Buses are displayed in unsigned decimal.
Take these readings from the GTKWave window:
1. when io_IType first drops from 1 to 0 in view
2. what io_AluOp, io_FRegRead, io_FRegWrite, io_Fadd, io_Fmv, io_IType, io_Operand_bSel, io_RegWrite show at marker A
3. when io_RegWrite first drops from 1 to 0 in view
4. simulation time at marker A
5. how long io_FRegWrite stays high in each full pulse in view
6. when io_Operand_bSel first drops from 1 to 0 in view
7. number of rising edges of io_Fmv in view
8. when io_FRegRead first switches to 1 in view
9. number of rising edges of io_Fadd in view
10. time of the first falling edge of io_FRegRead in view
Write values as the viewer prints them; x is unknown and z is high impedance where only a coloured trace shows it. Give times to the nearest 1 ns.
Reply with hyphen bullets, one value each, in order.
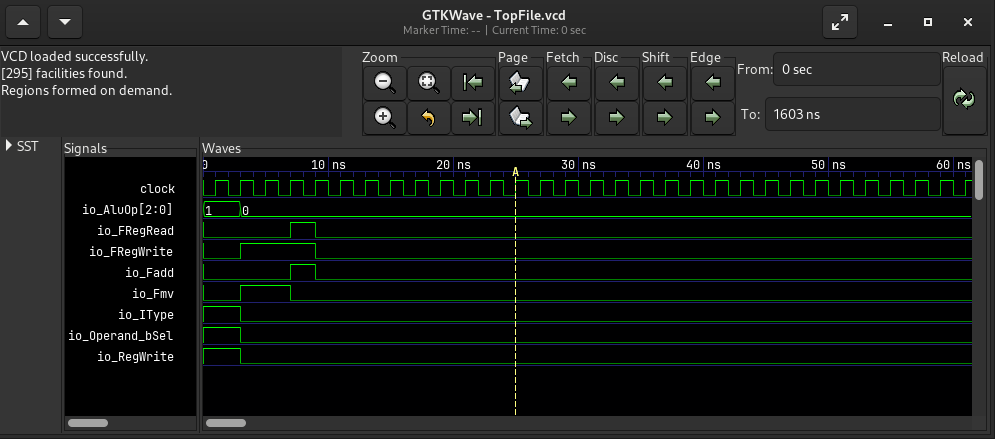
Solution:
- 3 ns
- io_AluOp=0, io_FRegRead=0, io_FRegWrite=0, io_Fadd=0, io_Fmv=0, io_IType=0, io_Operand_bSel=0, io_RegWrite=0
- 3 ns
- 25 ns
- 6 ns
- 3 ns
- 1
- 7 ns
- 1
- 9 ns
